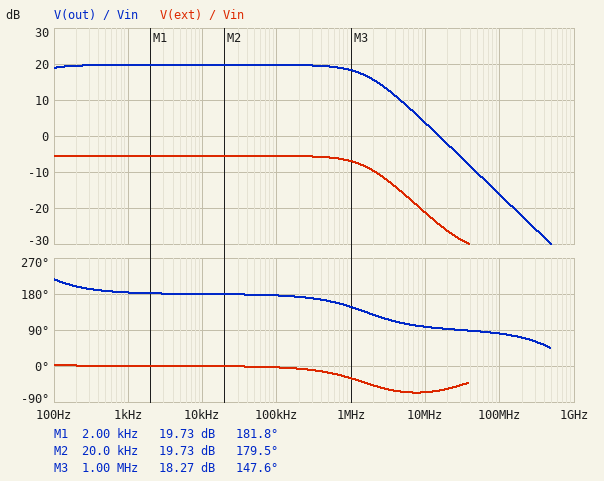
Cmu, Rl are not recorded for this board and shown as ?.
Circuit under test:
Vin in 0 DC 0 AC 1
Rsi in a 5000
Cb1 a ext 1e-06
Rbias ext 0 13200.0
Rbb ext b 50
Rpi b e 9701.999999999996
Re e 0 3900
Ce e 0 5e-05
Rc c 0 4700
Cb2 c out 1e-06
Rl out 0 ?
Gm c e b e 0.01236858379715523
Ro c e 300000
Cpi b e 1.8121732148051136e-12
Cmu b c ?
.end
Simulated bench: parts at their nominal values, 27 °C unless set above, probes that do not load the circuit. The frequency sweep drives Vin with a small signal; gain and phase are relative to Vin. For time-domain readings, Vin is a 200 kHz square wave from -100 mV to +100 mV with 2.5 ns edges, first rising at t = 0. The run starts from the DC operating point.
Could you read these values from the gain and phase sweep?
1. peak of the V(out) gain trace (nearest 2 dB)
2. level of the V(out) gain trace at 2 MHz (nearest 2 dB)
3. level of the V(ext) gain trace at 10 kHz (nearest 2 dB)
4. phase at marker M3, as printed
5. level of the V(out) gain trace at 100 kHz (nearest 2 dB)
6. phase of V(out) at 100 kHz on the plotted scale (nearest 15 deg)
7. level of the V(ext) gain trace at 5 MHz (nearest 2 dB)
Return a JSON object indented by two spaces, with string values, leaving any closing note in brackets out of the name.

{
  "peak of the V(out) gain trace": "20 dB",
  "level of the V(out) gain trace at 2 MHz": "16 dB",
  "level of the V(ext) gain trace at 10 kHz": "-6 dB",
  "phase at marker M3, as printed": "147.6 deg",
  "level of the V(out) gain trace at 100 kHz": "20 dB",
  "phase of V(out) at 100 kHz on the plotted scale": "180 deg",
  "level of the V(ext) gain trace at 5 MHz": "-16 dB"
}
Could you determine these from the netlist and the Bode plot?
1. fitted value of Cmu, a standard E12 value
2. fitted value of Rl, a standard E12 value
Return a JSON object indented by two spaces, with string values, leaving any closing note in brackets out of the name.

{
  "fitted value of Cmu, a standard E12 value": "1.8 pF",
  "fitted value of Rl, a standard E12 value": "2.2 kΩ"
}
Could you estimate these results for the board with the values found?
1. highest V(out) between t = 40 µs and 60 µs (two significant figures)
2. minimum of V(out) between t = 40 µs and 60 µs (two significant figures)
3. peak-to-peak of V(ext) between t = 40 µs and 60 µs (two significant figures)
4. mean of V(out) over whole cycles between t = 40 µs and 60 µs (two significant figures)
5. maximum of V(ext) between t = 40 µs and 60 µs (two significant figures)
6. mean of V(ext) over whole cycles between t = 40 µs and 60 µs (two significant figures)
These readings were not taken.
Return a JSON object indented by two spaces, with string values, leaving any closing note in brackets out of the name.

{
  "highest V(out) between t = 40 µs and 60 µs": "24 mV",
  "minimum of V(out) between t = 40 µs and 60 µs": "-1.9 V",
  "peak-to-peak of V(ext) between t = 40 µs and 60 µs": "110 mV",
  "mean of V(out) over whole cycles between t = 40 µs and 60 µs": "-950 mV",
  "maximum of V(ext) between t = 40 µs and 60 µs": "110 mV",
  "mean of V(ext) over whole cycles between t = 40 µs and 60 µs": "53 mV"
}
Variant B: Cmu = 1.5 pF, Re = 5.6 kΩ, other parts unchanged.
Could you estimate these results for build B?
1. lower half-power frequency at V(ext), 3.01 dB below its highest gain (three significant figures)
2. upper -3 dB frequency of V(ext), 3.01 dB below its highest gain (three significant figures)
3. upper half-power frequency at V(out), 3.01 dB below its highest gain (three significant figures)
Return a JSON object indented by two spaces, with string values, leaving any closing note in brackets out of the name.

{
  "lower half-power frequency at V(ext), 3.01 dB below its highest gain": "6.36 Hz",
  "upper -3 dB frequency of V(ext), 3.01 dB below its highest gain": "1.82 MHz",
  "upper half-power frequency at V(out), 3.01 dB below its highest gain": "1.88 MHz"
}
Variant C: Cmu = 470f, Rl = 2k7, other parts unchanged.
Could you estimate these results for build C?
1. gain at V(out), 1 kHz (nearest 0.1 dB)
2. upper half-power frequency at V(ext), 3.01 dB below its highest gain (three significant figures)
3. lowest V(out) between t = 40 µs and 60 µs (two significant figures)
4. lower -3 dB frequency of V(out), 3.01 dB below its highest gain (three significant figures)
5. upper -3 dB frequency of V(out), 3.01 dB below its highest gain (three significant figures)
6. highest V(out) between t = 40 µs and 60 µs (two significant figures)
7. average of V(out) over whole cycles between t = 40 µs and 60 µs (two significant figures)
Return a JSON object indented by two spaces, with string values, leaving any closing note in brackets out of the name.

{
  "gain at V(out), 1 kHz": "20.9 dB",
  "upper half-power frequency at V(ext), 3.01 dB below its highest gain": "4.63 MHz",
  "lowest V(out) between t = 40 µs and 60 µs": "-2.2 V",
  "lower -3 dB frequency of V(out), 3.01 dB below its highest gain": "47.6 Hz",
  "upper -3 dB frequency of V(out), 3.01 dB below its highest gain": "4.79 MHz",
  "highest V(out) between t = 40 µs and 60 µs": "27 mV",
  "average of V(out) over whole cycles between t = 40 µs and 60 µs": "-1.1 V"
}
